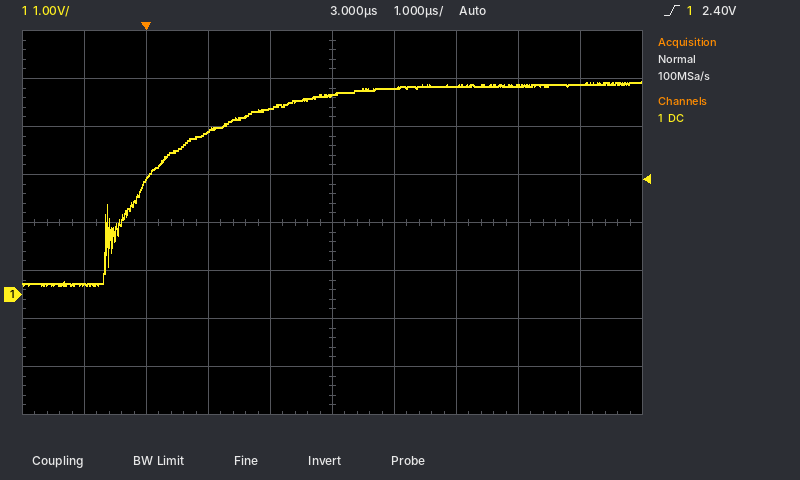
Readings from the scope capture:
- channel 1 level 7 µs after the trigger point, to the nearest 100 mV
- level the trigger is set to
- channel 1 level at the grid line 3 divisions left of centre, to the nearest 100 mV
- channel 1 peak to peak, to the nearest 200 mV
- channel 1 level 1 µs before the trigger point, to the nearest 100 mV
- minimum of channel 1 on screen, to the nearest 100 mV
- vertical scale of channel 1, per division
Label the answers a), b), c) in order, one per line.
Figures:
a) 4.4 V
b) 2.40 V
c) 2.4 V
d) 4.2 V
e) 200 mV
f) 200 mV
g) 1 V
